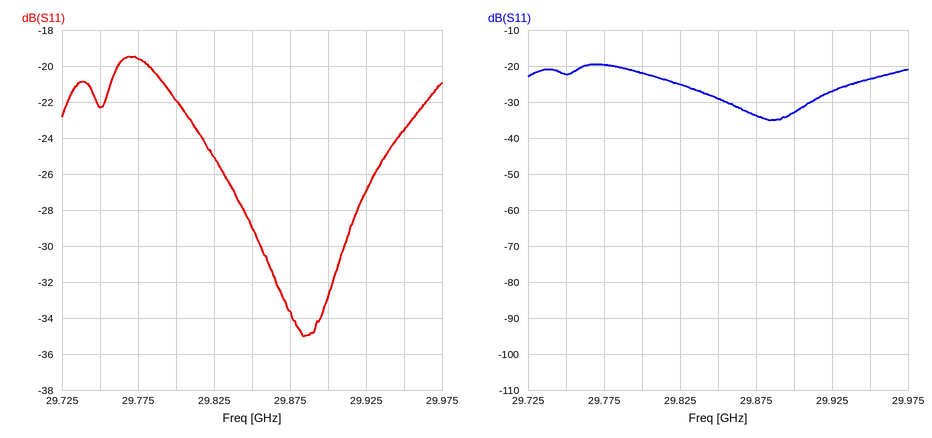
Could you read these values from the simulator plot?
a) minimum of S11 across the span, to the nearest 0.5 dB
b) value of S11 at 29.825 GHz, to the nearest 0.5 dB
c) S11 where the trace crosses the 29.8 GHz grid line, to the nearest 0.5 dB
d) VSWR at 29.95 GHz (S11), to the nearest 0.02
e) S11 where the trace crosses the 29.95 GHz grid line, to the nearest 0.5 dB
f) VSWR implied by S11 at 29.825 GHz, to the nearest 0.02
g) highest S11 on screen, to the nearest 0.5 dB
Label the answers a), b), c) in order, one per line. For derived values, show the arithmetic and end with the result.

a) -35.0 dB
b) -25.0 dB
c) -22.0 dB
d) |Γ| = 10^(-23.5/20) = 0.0668; VSWR = (1 + 0.0668)/(1 − 0.0668) ≈ 1.14
e) -23.5 dB
f) |Γ| = 10^(-25/20) = 0.0562; VSWR = (1 + 0.0562)/(1 − 0.0562) ≈ 1.12
g) -19.5 dB
